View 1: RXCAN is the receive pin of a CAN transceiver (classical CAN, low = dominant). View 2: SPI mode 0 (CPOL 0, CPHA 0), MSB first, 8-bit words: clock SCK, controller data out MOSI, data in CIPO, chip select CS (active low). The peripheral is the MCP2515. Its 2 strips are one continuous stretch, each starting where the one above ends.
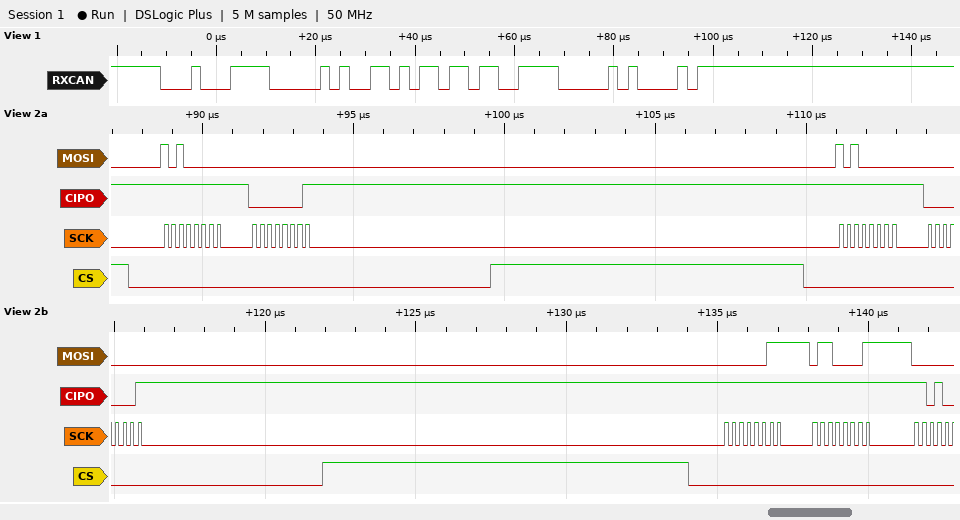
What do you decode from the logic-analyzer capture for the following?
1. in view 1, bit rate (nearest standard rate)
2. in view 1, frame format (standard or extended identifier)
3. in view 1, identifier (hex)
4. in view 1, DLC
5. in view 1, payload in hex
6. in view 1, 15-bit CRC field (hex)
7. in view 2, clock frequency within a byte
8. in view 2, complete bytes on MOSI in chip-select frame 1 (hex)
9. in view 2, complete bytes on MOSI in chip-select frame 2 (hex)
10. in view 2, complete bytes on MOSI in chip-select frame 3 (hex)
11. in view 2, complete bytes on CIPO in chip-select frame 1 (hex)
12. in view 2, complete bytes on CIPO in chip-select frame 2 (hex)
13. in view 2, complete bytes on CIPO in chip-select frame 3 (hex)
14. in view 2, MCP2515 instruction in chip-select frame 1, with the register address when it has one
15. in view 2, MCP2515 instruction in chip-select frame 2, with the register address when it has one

500 kbit/s
standard
0x11E
2
6B 6C
0x7810
4 MHz
A0 00
A0 00
03 61
FF 01
FF 01
FF FF
READ STATUS
READ STATUS
